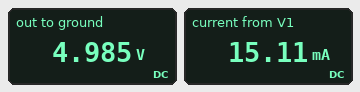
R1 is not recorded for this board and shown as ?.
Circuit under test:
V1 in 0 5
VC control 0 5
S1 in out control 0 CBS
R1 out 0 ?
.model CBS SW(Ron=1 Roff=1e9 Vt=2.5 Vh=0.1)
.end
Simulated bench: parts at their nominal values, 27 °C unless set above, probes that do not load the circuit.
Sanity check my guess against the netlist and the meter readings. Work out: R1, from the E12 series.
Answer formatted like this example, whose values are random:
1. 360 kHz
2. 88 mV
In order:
1. 330 Ω
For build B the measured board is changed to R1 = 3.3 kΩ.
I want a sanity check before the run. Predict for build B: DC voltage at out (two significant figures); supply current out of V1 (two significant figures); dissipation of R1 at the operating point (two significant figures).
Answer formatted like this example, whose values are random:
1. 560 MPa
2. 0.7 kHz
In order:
1. 5.0 V
2. 1.5 mA
3. 7.6 mW
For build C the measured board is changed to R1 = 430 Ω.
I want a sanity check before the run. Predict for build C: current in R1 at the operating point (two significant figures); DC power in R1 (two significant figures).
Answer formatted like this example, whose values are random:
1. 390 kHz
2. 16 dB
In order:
1. 12 mA
2. 58 mW
